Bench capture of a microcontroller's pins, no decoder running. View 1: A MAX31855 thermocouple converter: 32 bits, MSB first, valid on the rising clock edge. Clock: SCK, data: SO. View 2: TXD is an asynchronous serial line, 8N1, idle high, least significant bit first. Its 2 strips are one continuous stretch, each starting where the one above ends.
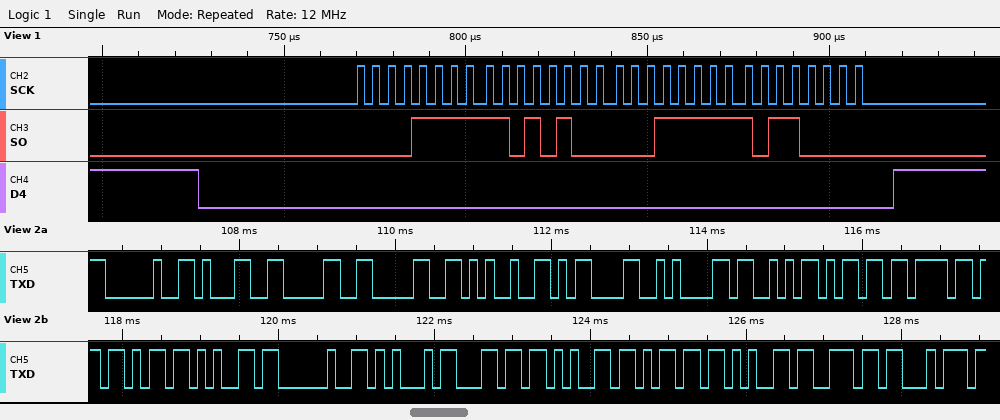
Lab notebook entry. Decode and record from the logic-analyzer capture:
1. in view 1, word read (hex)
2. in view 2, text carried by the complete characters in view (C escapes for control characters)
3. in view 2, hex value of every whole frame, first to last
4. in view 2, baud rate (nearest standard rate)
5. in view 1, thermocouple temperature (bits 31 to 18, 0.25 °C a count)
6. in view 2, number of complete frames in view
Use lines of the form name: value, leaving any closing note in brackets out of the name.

in view 1, word read: 0x0FD41FB0
in view 2, text carried by the complete characters in view: " 100%\r\nSmoke Element"
in view 2, hex value of every whole frame, first to last: 20 31 30 30 25 0D 0A 53 6D 6F 6B 65 20 45 6C 65 6D 65 6E 74
in view 2, baud rate: 9600 baud
in view 1, thermocouple temperature: 253.25 °C
in view 2, number of complete frames in view: 20
